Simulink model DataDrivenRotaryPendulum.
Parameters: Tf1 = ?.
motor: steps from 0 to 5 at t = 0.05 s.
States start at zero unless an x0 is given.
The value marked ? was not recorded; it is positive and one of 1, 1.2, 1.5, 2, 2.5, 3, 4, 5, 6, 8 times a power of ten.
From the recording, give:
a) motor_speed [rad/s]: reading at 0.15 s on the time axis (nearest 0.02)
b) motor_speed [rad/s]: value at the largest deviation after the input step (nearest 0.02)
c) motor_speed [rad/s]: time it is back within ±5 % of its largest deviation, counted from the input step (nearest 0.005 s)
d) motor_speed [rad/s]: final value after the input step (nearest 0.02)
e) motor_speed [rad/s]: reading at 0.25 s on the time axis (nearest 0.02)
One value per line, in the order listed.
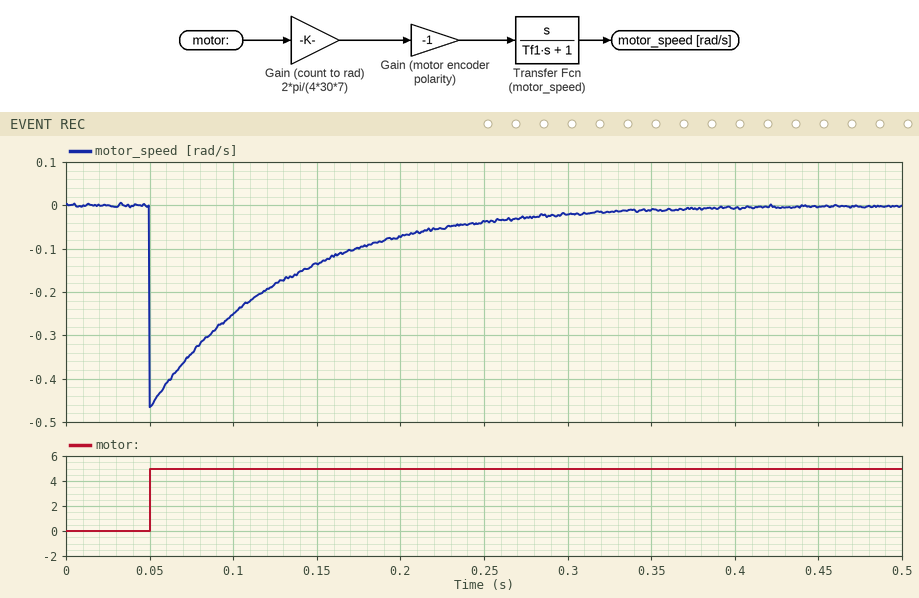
-0.14
-0.46
0.240 s
0.00
-0.04
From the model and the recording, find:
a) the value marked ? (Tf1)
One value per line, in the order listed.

0.08
